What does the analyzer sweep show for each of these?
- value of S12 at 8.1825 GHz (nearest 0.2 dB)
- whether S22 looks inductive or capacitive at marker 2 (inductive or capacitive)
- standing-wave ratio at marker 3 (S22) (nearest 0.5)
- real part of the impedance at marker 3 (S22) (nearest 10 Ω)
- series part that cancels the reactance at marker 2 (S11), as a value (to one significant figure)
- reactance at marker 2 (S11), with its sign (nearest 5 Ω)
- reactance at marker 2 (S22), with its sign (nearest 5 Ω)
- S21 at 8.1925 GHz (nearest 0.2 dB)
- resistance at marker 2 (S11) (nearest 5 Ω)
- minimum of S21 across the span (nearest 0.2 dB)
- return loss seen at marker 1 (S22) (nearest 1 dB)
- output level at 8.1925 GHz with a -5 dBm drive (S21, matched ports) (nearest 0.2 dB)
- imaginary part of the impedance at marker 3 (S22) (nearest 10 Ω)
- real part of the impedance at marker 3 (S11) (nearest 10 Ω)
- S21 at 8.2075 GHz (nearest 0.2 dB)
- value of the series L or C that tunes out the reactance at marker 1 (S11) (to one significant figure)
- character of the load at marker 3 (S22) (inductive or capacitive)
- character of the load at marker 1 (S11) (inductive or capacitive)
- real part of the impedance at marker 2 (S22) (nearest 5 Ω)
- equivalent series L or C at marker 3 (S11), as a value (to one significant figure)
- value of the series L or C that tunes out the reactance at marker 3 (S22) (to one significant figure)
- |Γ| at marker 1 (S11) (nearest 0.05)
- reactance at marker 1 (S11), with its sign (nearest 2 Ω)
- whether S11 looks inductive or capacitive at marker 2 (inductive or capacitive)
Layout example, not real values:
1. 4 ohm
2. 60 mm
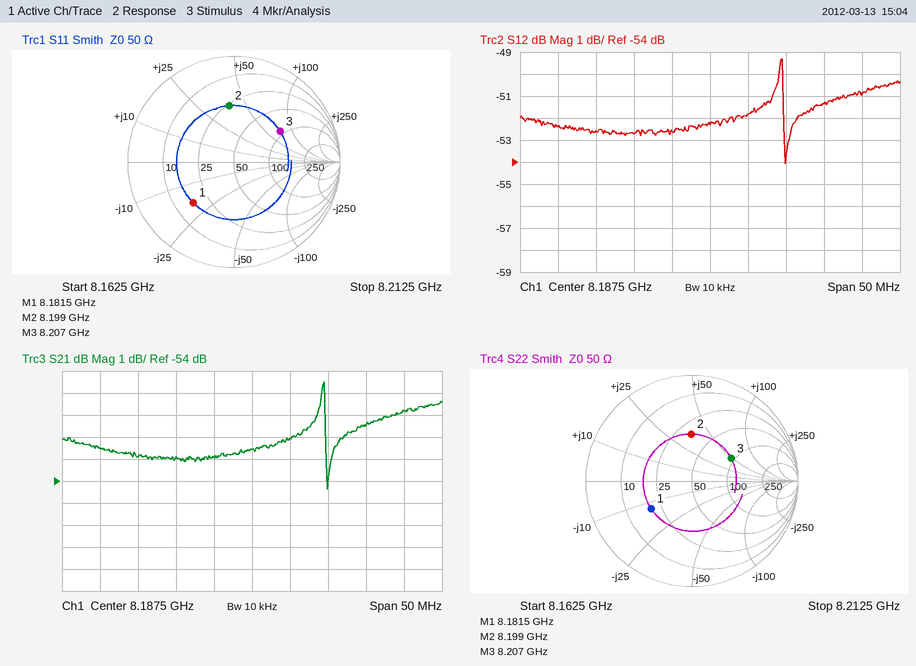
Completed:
1. -52.6 dB
2. inductive
3. 2.5
4. 90 Ω
5. 500 fF
6. +40 Ω
7. +35 Ω
8. -52.0 dB
9. 25 Ω
10. -54.4 dB
11. 7 dB
12. -57.0 dBm
13. +50 Ω
14. 90 Ω
15. -50.8 dB
16. 400 pH
17. inductive
18. capacitive
19. 35 Ω
20. 1 nH
21. 400 fF
22. 0.55
23. -18 Ω
24. inductive
